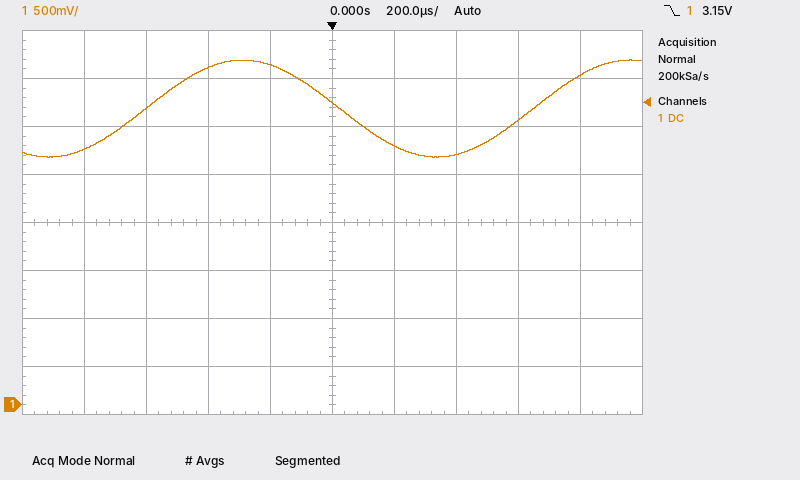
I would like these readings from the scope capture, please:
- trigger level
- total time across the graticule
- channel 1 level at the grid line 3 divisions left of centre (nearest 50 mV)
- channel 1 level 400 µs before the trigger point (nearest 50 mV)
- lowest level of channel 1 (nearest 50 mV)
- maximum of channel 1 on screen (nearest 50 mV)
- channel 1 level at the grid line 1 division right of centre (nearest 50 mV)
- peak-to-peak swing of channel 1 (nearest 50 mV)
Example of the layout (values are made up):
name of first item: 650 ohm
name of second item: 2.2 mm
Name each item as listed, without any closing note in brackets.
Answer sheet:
trigger level: 3.15 V
total time across the graticule: 2 ms
channel 1 level at the grid line 3 divisions left of centre: 3.10 V
channel 1 level 400 µs before the trigger point: 3.50 V
lowest level of channel 1: 2.60 V
maximum of channel 1 on screen: 3.60 V
channel 1 level at the grid line 1 division right of centre: 2.70 V
peak-to-peak swing of channel 1: 1.00 V
